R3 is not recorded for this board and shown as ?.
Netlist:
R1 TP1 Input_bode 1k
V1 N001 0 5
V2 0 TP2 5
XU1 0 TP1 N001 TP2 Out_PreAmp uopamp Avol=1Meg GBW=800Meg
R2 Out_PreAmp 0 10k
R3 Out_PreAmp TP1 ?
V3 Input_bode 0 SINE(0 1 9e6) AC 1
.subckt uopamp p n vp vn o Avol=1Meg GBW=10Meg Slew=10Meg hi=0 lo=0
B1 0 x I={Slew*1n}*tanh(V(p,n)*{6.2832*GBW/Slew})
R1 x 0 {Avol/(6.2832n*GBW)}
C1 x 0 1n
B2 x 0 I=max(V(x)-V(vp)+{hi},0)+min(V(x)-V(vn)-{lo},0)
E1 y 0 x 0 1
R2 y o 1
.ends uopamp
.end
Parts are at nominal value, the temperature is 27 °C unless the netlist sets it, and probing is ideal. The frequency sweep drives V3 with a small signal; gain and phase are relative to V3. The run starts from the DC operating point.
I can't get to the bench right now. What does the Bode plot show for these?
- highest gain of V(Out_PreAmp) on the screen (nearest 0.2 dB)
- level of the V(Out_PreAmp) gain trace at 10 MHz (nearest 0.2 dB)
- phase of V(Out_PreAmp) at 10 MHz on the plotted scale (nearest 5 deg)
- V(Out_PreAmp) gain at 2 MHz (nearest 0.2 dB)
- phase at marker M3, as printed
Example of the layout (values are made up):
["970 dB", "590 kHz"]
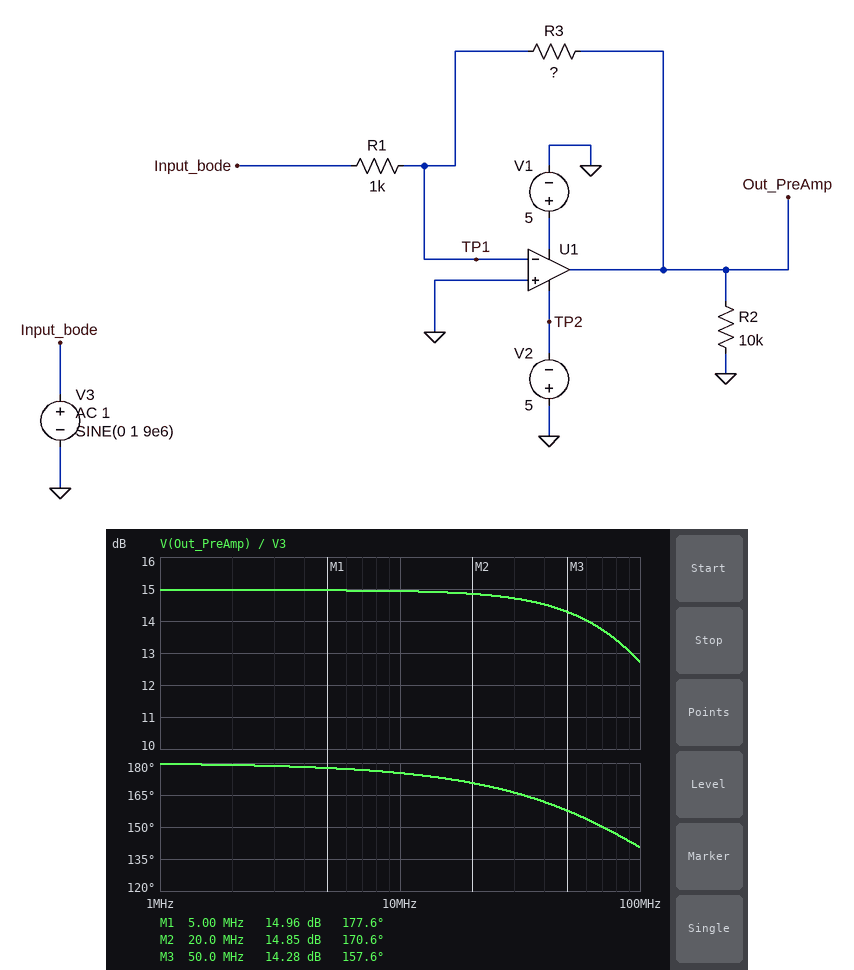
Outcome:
["15.0 dB", "15.0 dB", "175 deg", "15.0 dB", "157.6 deg"]
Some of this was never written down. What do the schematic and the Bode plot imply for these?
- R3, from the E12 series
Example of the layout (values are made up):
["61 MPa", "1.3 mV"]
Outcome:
["5.6 kΩ"]
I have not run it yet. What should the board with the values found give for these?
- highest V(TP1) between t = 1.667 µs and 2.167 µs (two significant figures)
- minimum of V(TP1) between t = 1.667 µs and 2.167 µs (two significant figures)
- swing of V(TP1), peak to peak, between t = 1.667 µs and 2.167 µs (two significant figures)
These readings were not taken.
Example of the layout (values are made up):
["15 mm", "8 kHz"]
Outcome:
["840 mV", "-850 mV", "1.7 V"]
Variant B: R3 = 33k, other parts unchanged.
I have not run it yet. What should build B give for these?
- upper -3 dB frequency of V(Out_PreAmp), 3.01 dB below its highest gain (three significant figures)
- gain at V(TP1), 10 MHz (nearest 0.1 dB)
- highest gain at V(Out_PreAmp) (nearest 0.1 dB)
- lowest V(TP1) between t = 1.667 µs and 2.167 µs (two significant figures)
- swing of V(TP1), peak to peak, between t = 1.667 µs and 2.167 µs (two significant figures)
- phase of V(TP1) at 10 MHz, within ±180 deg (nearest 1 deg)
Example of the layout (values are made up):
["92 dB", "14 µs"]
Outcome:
["23.5 MHz", "-8.4 dB", "30.4 dB", "-980 mV", "1.9 V", "67 deg"]
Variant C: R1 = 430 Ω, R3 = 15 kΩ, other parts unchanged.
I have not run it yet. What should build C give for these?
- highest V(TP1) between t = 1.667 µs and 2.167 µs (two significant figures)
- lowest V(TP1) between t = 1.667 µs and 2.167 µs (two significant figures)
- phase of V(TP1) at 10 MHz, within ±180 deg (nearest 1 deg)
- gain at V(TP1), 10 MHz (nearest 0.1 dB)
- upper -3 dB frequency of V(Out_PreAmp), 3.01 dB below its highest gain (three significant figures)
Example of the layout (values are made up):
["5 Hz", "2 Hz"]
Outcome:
["970 mV", "-980 mV", "66 deg", "-8.0 dB", "22.3 MHz"]
